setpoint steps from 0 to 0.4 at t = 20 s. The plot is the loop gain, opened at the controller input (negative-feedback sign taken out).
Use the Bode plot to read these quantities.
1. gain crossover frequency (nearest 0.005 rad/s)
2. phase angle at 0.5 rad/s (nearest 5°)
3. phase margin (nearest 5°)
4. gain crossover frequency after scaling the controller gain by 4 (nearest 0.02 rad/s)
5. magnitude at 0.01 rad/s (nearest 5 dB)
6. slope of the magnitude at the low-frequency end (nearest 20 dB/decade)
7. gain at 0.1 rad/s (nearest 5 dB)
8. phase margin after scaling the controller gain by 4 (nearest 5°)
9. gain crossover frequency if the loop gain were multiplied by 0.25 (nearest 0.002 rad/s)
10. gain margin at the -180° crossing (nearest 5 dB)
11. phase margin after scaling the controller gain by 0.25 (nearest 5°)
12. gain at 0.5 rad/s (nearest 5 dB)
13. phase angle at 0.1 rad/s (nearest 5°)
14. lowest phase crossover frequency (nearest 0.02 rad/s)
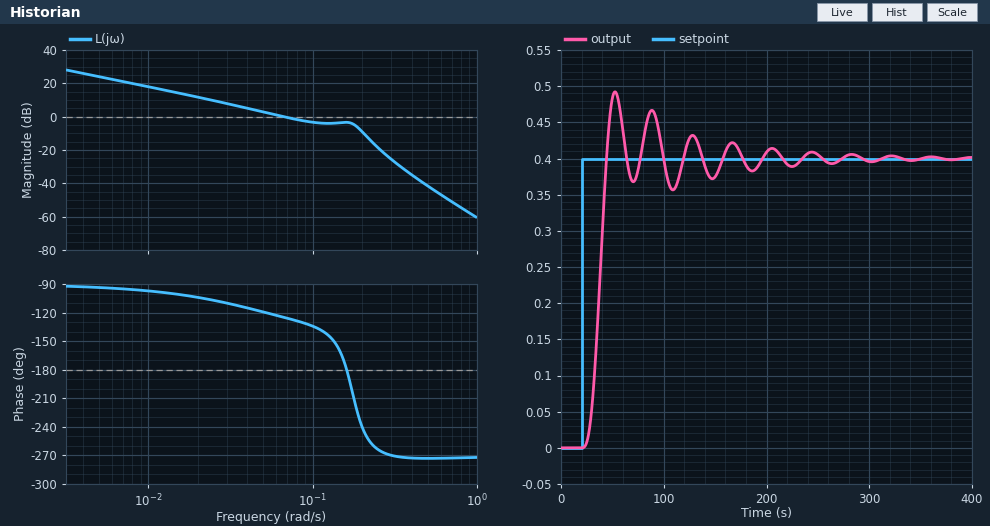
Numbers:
0.065 rad/s
-275°
55°
0.22 rad/s
20 dB
-20 dB/decade
-5 dB
-70°
0.020 rad/s
5 dB
75°
-40 dB
-135°
0.16 rad/s
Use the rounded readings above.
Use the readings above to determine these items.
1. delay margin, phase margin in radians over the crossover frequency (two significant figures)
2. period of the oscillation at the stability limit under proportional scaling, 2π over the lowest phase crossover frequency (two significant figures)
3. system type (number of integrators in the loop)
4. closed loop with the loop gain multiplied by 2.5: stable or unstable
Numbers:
15 s
39 s
1
unstable
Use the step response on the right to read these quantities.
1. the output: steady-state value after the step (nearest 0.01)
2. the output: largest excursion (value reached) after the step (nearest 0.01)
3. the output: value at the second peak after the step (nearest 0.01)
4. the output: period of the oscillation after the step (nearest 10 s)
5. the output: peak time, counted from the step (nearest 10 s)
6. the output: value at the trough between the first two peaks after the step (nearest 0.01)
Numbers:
0.40
0.49
0.47
40 s
30 s
0.37
